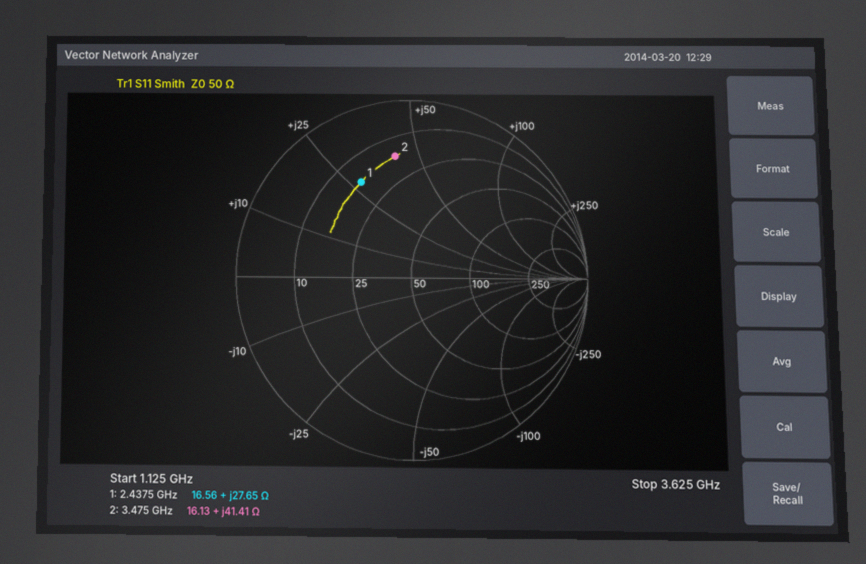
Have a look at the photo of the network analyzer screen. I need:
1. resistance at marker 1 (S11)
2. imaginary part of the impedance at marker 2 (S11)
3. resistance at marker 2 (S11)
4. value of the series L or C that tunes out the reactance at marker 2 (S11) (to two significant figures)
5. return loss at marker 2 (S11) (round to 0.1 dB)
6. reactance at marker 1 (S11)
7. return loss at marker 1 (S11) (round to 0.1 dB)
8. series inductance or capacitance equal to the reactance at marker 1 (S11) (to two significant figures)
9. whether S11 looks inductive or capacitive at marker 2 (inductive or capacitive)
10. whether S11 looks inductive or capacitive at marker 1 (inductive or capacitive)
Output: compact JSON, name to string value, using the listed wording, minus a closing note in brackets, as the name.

{"resistance at marker 1": "16.56 Ω", "imaginary part of the impedance at marker 2": "+41.41 Ω", "resistance at marker 2": "16.13 Ω", "value of the series L or C that tunes out the reactance at marker 2 (S11)": "1.1 pF", "return loss at marker 2 (S11)": "3.3 dB", "reactance at marker 1": "+27.65 Ω", "return loss at marker 1 (S11)": "4.4 dB", "series inductance or capacitance equal to the reactance at marker 1 (S11)": "1.8 nH", "whether S11 looks inductive or capacitive at marker 2": "inductive", "whether S11 looks inductive or capacitive at marker 1": "inductive"}
